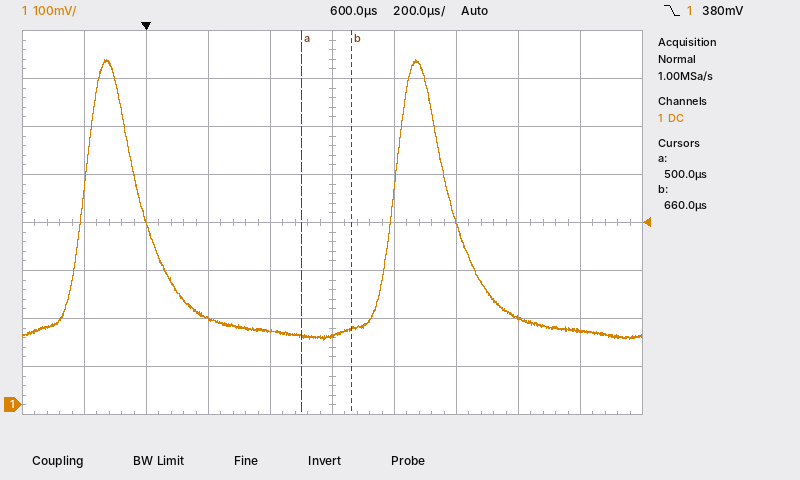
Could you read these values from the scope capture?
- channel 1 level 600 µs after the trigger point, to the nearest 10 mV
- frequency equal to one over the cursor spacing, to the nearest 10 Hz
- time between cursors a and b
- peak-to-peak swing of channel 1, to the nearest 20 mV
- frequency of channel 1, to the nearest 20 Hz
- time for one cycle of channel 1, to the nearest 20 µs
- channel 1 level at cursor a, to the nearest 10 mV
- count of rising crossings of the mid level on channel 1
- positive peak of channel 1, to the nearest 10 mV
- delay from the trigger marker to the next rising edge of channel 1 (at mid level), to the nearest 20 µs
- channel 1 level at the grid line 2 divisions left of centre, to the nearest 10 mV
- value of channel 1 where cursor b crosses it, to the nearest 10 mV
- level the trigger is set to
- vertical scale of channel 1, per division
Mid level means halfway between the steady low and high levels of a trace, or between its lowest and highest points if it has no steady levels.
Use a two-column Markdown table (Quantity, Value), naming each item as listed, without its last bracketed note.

| Quantity | Value |
|---|---|
| channel 1 level 600 µs after the trigger point, to the nearest 10 mV | 140 mV |
| frequency equal to one over the cursor spacing, to the nearest 10 Hz | 6.25 kHz |
| time between cursors a and b | 160 µs |
| peak-to-peak swing of channel 1, to the nearest 20 mV | 580 mV |
| frequency of channel 1, to the nearest 20 Hz | 1.00 kHz |
| time for one cycle of channel 1, to the nearest 20 µs | 1.00 ms |
| channel 1 level at cursor a, to the nearest 10 mV | 140 mV |
| count of rising crossings of the mid level on channel 1 | 2 |
| positive peak of channel 1, to the nearest 10 mV | 720 mV |
| delay from the trigger marker to the next rising edge of channel 1 (at mid level), to the nearest 20 µs | 800 µs |
| channel 1 level at the grid line 2 divisions left of centre, to the nearest 10 mV | 180 mV |
| value of channel 1 where cursor b crosses it, to the nearest 10 mV | 160 mV |
| level the trigger is set to | 380 mV |
| vertical scale of channel 1, per division | 100 mV |
